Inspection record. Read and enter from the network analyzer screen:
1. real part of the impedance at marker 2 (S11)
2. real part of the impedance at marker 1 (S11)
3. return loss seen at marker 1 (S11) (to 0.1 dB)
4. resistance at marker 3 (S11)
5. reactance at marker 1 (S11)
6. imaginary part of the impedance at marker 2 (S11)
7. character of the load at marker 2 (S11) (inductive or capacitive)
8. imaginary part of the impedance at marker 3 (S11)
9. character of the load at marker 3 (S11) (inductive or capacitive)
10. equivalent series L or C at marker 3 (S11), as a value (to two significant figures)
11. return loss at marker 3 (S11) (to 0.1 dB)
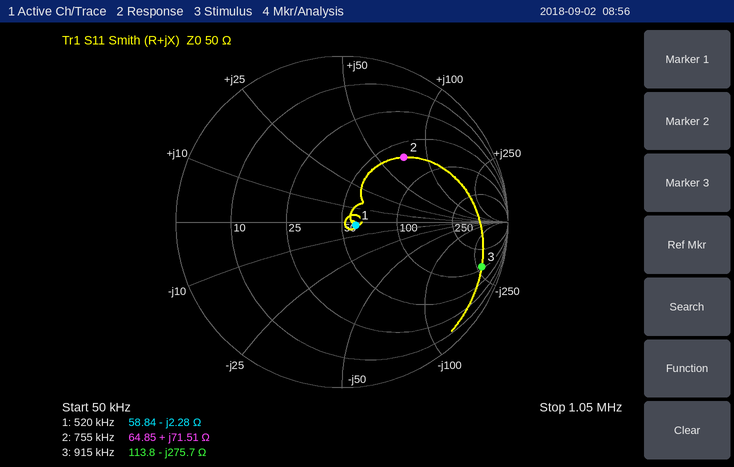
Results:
64.85 Ω
58.84 Ω
21.5 dB
113.8 Ω
-2.28 Ω
+71.51 Ω
inductive
-275.7 Ω
capacitive
630 pF
1.1 dB
